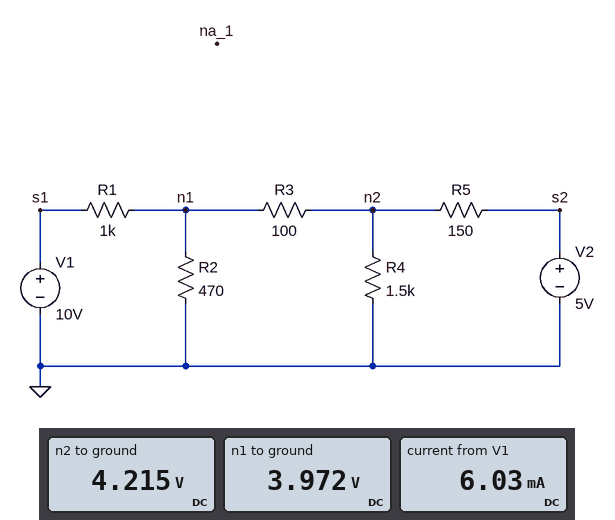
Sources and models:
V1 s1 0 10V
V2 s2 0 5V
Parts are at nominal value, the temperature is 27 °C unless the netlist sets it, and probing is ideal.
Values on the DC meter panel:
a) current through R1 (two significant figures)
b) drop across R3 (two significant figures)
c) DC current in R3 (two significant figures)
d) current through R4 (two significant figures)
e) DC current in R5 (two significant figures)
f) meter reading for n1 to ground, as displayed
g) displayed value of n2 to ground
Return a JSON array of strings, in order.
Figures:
["6.0 mA", "240 mV", "2.4 mA", "2.8 mA", "5.2 mA", "3.972 V", "4.215 V"]
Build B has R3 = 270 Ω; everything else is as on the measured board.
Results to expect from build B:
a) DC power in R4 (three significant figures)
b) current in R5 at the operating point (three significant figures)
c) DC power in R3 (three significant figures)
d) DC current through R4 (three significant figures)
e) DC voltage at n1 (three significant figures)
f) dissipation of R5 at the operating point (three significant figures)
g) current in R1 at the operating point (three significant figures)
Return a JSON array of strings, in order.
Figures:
["12.3 mW", "4.72 mA", "931 µW", "2.86 mA", "3.79 V", "3.34 mW", "6.21 mA"]
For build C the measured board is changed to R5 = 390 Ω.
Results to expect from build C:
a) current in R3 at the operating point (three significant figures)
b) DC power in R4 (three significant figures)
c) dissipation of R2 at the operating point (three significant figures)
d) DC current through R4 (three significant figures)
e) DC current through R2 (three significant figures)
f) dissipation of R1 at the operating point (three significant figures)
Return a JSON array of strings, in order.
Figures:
["1.06 mA", "8.84 mW", "26.6 mW", "2.43 mA", "7.52 mA", "41.8 mW"]
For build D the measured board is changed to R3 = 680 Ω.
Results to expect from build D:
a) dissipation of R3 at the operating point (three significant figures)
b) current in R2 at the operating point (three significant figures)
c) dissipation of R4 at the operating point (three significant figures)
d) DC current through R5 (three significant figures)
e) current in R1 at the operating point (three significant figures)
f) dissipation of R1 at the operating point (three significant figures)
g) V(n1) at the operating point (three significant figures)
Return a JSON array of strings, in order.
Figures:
["958 µW", "7.61 mA", "12.8 mW", "4.11 mA", "6.42 mA", "41.3 mW", "3.58 V"]
